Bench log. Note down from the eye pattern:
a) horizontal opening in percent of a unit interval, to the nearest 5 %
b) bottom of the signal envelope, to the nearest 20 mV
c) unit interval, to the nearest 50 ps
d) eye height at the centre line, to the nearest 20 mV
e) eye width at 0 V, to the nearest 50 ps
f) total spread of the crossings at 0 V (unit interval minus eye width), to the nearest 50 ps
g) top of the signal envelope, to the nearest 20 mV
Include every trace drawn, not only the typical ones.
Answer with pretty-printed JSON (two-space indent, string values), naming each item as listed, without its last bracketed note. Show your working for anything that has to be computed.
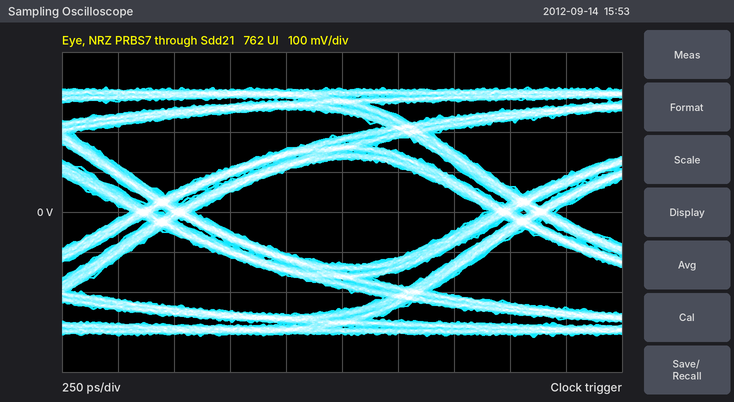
{
  "horizontal opening in percent of a unit interval, to the nearest 5 %": "1.30 ns / 1.60 ns ≈ 81.2 %, so 80 % to the nearest 5 %",
  "bottom of the signal envelope, to the nearest 20 mV": "-320 mV",
  "unit interval, to the nearest 50 ps": "1.60 ns",
  "eye height at the centre line, to the nearest 20 mV": "260 mV",
  "eye width at 0 V, to the nearest 50 ps": "1.30 ns",
  "total spread of the crossings at 0 V (unit interval minus eye width), to the nearest 50 ps": "300 ps",
  "top of the signal envelope, to the nearest 20 mV": "320 mV"
}
